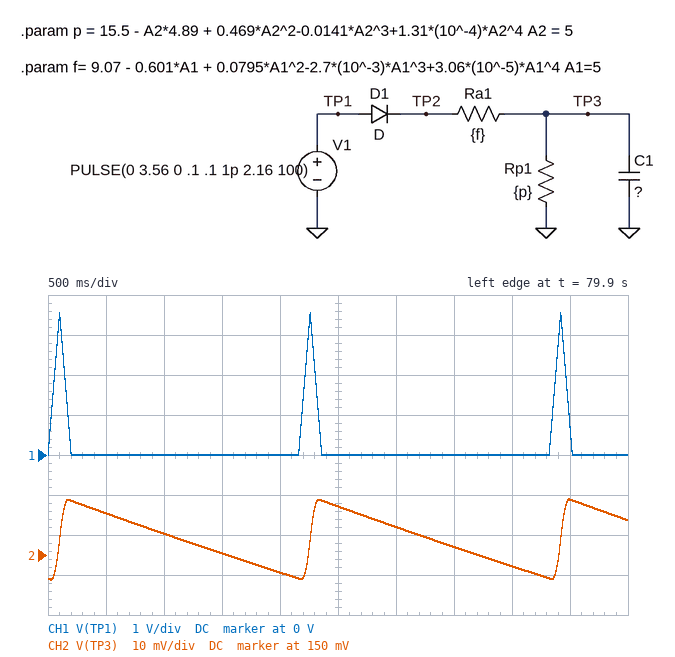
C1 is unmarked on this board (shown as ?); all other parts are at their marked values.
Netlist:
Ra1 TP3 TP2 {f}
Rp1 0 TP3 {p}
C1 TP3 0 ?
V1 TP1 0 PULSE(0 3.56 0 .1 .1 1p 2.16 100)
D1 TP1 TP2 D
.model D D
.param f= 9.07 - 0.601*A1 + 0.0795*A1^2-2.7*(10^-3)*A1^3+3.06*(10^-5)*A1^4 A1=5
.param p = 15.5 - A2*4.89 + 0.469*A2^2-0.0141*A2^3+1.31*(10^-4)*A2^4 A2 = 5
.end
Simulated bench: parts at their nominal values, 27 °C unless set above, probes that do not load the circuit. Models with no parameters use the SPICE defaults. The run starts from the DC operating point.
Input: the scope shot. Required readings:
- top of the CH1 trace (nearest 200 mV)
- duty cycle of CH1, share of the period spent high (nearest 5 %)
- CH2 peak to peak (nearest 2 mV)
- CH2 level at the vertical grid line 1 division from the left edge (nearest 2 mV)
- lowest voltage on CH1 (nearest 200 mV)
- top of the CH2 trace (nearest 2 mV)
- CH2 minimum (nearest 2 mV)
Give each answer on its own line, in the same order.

3.6 V
5 %
20 mV
160 mV
0 V
164 mV
144 mV
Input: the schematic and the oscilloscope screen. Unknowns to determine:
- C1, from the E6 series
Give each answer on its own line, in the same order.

1 F
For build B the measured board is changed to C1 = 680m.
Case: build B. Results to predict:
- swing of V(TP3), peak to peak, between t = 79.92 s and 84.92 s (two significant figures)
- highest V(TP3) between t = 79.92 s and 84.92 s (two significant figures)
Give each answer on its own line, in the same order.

29 mV
170 mV
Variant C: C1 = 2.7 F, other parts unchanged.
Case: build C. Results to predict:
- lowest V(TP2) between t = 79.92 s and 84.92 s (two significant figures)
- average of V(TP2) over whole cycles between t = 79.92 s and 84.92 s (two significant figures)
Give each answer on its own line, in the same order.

130 mV
230 mV
